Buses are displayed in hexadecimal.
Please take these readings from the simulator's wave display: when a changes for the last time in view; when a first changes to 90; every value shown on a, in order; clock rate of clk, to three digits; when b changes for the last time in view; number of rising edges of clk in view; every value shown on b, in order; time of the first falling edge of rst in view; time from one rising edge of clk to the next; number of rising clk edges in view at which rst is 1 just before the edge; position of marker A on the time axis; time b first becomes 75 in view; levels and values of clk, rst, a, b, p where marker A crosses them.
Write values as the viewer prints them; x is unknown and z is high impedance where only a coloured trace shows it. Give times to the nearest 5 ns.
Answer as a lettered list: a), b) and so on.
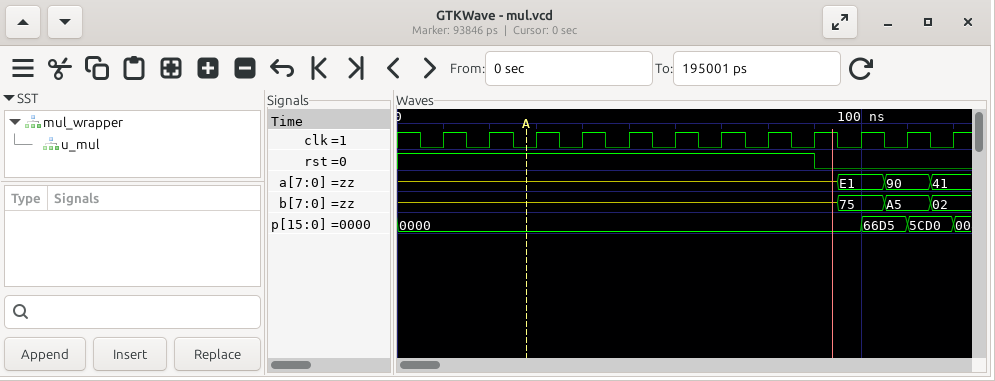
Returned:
a) 115 ns
b) 105 ns
c) z, E1, 90, 41
d) 100 MHz
e) 115 ns
f) 12
g) z, 75, A5, 02
h) 90 ns
i) 10 ns
j) 9
k) 30 ns
l) 95 ns
m) clk=0, rst=1, a=z, b=z, p=0000
